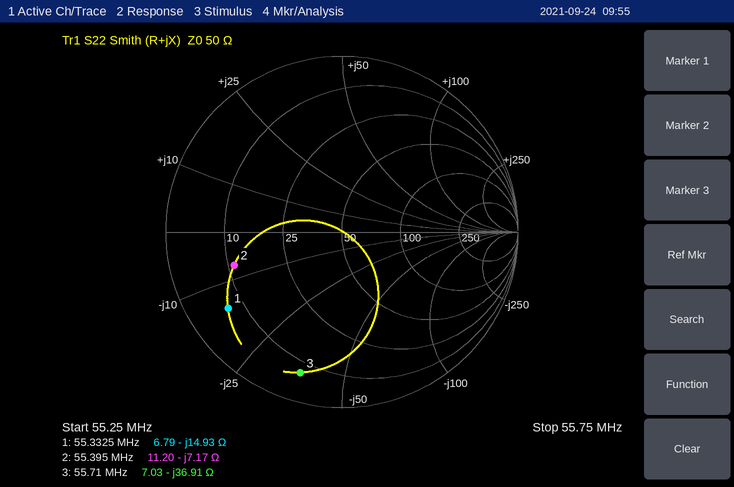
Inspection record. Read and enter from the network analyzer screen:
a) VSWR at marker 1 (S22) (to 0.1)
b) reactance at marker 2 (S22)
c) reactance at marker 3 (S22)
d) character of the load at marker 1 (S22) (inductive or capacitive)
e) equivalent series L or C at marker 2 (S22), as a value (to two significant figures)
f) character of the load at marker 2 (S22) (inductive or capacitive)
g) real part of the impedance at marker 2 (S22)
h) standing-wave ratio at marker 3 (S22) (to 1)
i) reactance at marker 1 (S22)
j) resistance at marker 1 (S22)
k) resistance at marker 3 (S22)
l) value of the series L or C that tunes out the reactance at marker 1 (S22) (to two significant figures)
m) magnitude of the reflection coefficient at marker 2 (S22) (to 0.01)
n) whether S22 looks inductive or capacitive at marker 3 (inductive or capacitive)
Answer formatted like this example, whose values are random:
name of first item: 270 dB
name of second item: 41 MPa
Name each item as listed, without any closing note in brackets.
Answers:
VSWR at marker 1 (S22): 8.0
reactance at marker 2: -7.17 Ω
reactance at marker 3: -36.91 Ω
character of the load at marker 1 (S22): capacitive
equivalent series L or C at marker 2 (S22), as a value: 400 pF
character of the load at marker 2 (S22): capacitive
real part of the impedance at marker 2: 11.20 Ω
standing-wave ratio at marker 3 (S22): 11
reactance at marker 1: -14.93 Ω
resistance at marker 1: 6.79 Ω
resistance at marker 3: 7.03 Ω
value of the series L or C that tunes out the reactance at marker 1 (S22): 43 nH
magnitude of the reflection coefficient at marker 2 (S22): 0.64
whether S22 looks inductive or capacitive at marker 3: capacitive
